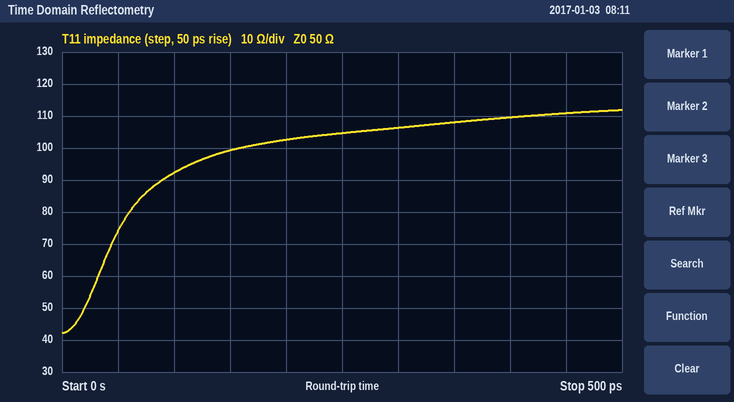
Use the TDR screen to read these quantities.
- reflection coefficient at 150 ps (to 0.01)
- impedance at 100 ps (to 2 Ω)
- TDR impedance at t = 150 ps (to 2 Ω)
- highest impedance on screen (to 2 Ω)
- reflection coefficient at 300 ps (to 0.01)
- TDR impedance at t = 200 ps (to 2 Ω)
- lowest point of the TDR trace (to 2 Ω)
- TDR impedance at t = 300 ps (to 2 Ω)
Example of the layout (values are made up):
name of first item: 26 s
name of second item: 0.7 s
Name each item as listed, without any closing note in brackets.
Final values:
reflection coefficient at 150 ps: +0.33
impedance at 100 ps: 92 Ω
TDR impedance at t = 150 ps: 100 Ω
highest impedance on screen: 112 Ω
reflection coefficient at 300 ps: +0.36
TDR impedance at t = 200 ps: 102 Ω
lowest point of the TDR trace: 42 Ω
TDR impedance at t = 300 ps: 106 Ω
